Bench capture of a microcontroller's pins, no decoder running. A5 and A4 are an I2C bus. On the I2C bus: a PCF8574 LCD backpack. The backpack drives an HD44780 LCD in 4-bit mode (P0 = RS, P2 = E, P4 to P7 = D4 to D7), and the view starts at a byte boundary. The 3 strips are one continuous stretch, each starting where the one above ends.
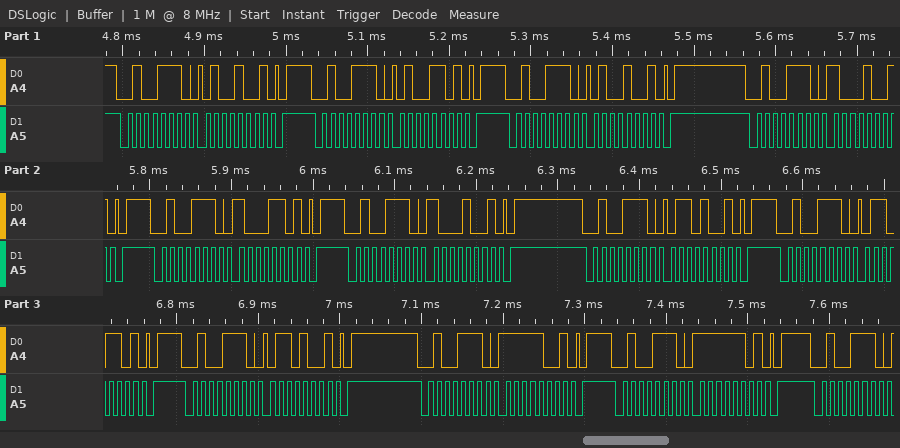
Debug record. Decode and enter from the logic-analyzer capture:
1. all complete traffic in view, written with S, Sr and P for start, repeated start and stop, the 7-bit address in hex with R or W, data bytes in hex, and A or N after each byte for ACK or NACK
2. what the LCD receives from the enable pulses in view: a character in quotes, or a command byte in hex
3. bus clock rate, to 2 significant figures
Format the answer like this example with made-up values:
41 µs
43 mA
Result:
S 27W A 49 A P S 27W A 4D A P S 27W A 49 A P S 27W A 89 A P S 27W A 8D A P S 27W A 89 A P S 27W A 69 A P S 27W A 6D A P S 27W A 69 A P S 27W A F9 A P S 27W A FD A P S 27W A
'H'
100 kHz
